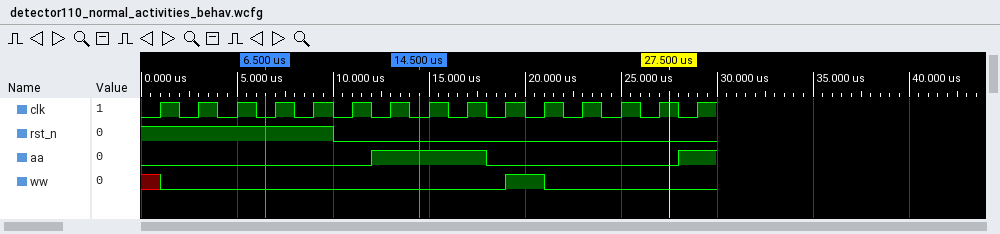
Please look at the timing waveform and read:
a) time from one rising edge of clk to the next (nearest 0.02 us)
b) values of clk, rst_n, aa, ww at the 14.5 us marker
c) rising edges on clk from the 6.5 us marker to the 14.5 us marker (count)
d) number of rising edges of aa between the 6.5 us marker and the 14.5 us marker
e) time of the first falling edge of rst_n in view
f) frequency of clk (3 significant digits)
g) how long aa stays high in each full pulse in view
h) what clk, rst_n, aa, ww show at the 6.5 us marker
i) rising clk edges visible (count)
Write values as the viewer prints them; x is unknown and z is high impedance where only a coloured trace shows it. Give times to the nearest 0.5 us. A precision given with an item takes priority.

2 us
clk=0, rst_n=0, aa=1, ww=0
4
1
10 us
500 kHz
6 us
clk=0, rst_n=1, aa=0, ww=0
15
